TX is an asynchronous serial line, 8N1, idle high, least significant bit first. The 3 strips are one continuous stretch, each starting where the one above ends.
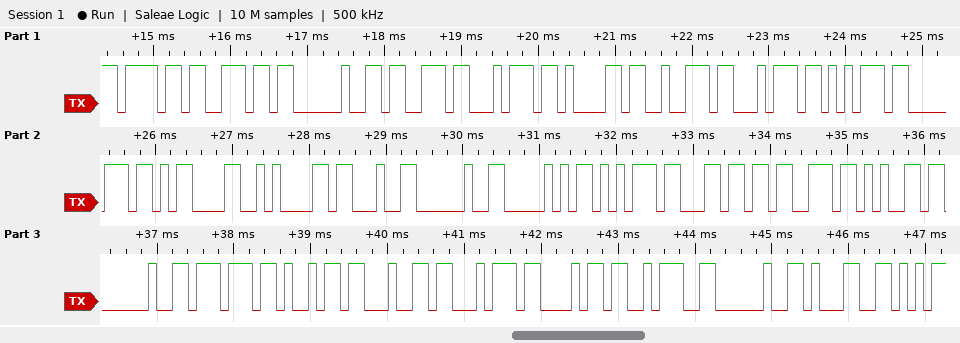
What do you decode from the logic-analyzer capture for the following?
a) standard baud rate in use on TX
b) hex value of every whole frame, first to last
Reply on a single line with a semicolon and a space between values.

9600 baud; 6F 6E 20 73 74 61 72 74 75 70 0D 0A 23 20 50 75 6C 73 65 20 77 69 64 74 68 3A 20 31
